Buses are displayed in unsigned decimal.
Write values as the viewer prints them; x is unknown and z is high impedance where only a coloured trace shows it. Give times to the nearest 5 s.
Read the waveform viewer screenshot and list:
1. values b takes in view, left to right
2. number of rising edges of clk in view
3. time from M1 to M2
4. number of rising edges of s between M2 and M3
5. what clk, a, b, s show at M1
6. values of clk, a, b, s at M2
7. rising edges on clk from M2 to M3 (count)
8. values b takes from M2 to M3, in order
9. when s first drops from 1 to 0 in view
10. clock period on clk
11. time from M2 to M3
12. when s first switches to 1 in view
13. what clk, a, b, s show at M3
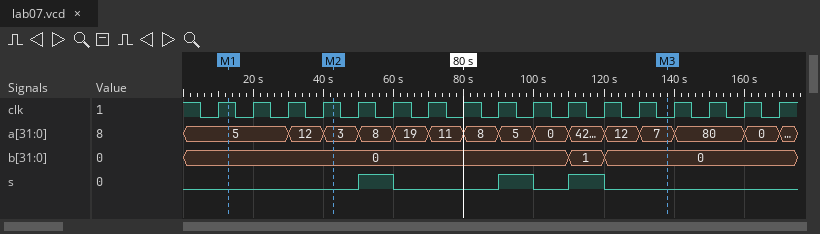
0, 1, 0
17
30 s
3
clk=1, a=5, b=0, s=0
clk=1, a=3, b=0, s=0
9
0, 1, 0
60 s
10 s
95 s
50 s
clk=0, a=7, b=0, s=0
